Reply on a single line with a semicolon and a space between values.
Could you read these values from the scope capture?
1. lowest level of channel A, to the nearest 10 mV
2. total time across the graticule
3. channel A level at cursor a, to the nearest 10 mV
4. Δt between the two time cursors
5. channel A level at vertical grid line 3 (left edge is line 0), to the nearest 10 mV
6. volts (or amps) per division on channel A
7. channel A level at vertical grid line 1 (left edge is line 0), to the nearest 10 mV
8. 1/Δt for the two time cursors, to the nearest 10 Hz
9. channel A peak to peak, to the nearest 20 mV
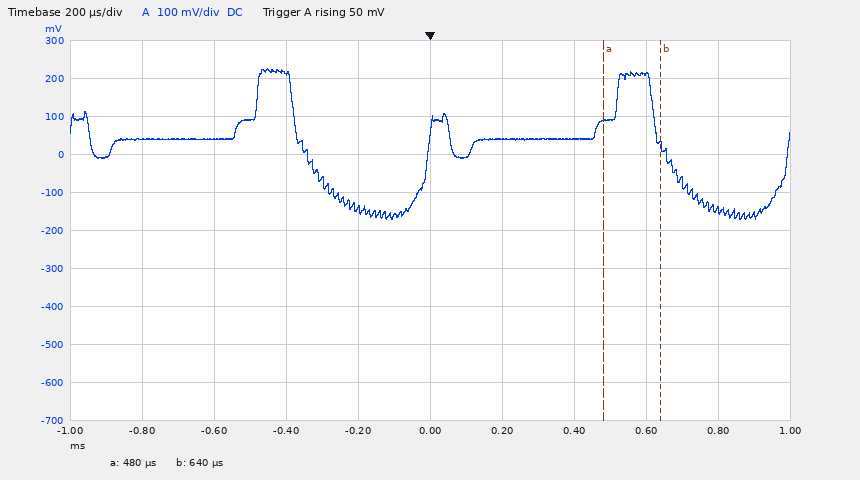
-170 mV; 2 ms; 90 mV; 160 µs; 210 mV; 100 mV; 40 mV; 6.25 kHz; 400 mV
